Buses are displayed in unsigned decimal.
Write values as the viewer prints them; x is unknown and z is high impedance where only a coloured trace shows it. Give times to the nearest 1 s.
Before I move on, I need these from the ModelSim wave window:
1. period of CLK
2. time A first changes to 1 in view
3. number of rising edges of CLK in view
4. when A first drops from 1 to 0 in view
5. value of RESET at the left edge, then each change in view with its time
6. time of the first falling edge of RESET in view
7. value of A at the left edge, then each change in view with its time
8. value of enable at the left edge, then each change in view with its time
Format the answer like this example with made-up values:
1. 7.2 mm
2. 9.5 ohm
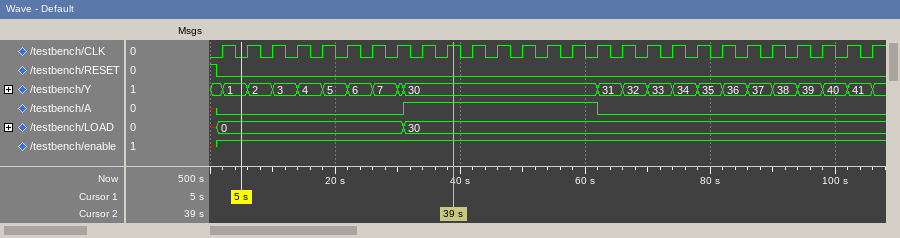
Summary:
1. 4 s
2. 31 s
3. 27
4. 62 s
5. 1, 0 at 1 s
6. 1 s
7. x, 0 at 1 s, 1 at 31 s, 0 at 62 s
8. x, 1 at 1 s
